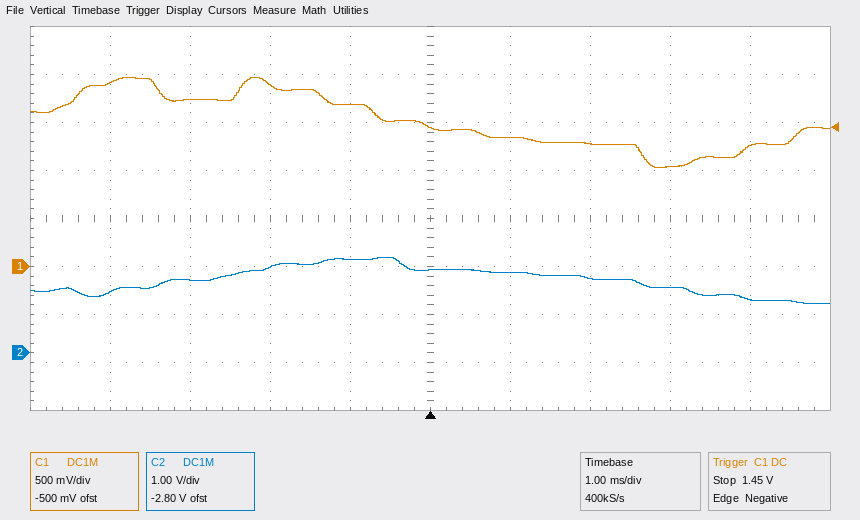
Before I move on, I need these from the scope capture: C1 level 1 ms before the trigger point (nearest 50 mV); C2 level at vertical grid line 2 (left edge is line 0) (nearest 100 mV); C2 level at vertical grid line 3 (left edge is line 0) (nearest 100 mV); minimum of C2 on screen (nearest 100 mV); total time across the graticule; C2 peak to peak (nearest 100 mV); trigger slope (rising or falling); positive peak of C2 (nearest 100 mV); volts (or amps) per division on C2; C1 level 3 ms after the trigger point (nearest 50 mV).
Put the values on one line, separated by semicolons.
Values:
1.70 V; 1.5 V; 1.8 V; 1.0 V; 10 ms; 1.0 V; falling; 2.0 V; 1 V; 1.05 V
